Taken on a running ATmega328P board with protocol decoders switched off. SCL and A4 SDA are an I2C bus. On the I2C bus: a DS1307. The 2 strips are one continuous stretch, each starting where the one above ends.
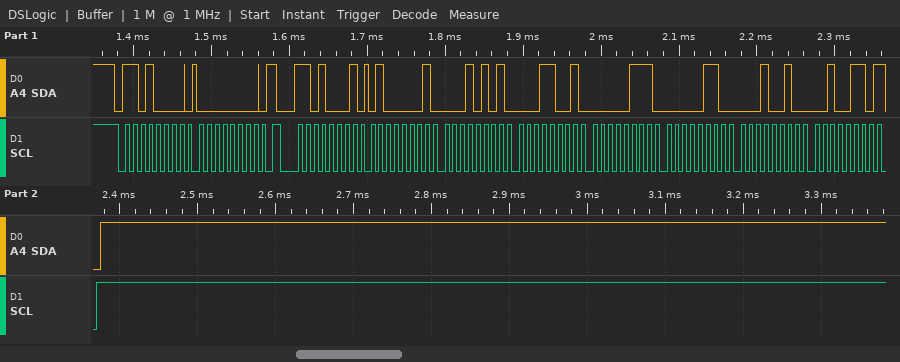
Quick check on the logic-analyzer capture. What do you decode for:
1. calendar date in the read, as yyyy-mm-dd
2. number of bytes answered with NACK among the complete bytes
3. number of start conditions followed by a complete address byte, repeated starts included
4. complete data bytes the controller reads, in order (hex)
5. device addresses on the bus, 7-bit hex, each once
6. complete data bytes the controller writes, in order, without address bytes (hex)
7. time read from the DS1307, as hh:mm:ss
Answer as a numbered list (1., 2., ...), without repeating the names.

1. 2026-12-06
2. 1
3. 2
4. 41 15 19 07 06 12 26
5. 0x68
6. 00
7. 19:15:41
